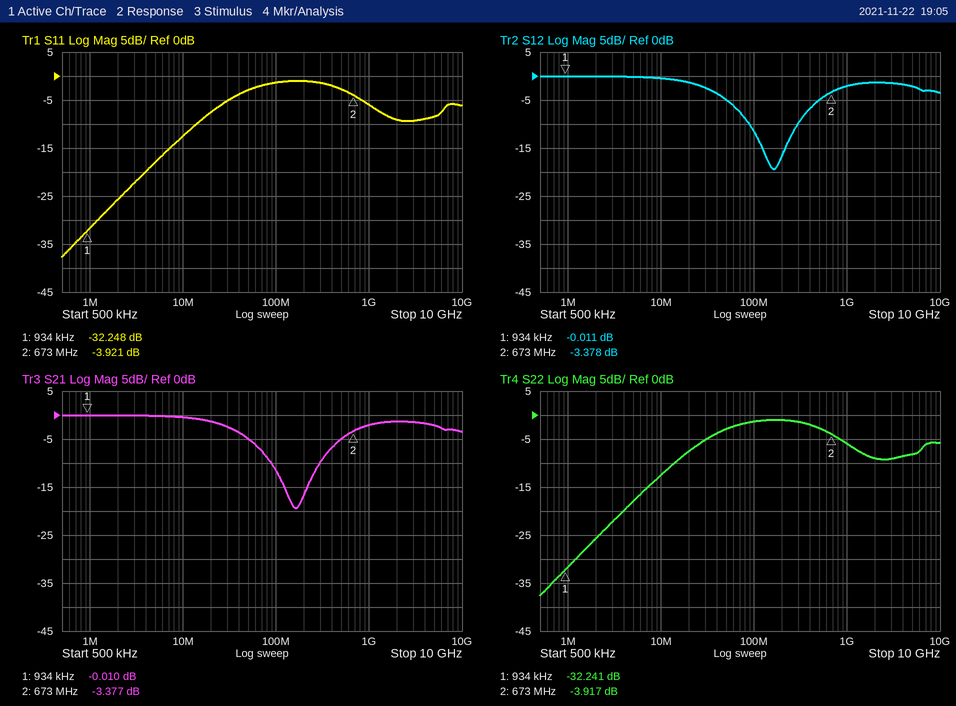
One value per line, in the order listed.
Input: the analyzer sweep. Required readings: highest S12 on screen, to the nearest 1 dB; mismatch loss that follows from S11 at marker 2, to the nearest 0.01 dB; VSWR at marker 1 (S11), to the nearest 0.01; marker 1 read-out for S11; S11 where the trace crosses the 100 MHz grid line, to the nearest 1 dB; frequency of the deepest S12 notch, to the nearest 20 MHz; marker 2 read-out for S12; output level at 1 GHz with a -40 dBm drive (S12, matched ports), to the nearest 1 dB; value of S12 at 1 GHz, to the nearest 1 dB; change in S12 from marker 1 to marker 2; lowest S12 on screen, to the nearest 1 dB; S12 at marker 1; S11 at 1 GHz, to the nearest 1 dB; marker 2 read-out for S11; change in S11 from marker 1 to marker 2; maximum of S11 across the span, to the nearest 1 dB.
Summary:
0 dB
2.26 dB
1.05
-32.248 dB
-1 dB
160 MHz
-3.378 dB
-42 dBm
-2 dB
-3.367 dB
-19 dB
-0.011 dB
-6 dB
-3.921 dB
28.327 dB
-1 dB
